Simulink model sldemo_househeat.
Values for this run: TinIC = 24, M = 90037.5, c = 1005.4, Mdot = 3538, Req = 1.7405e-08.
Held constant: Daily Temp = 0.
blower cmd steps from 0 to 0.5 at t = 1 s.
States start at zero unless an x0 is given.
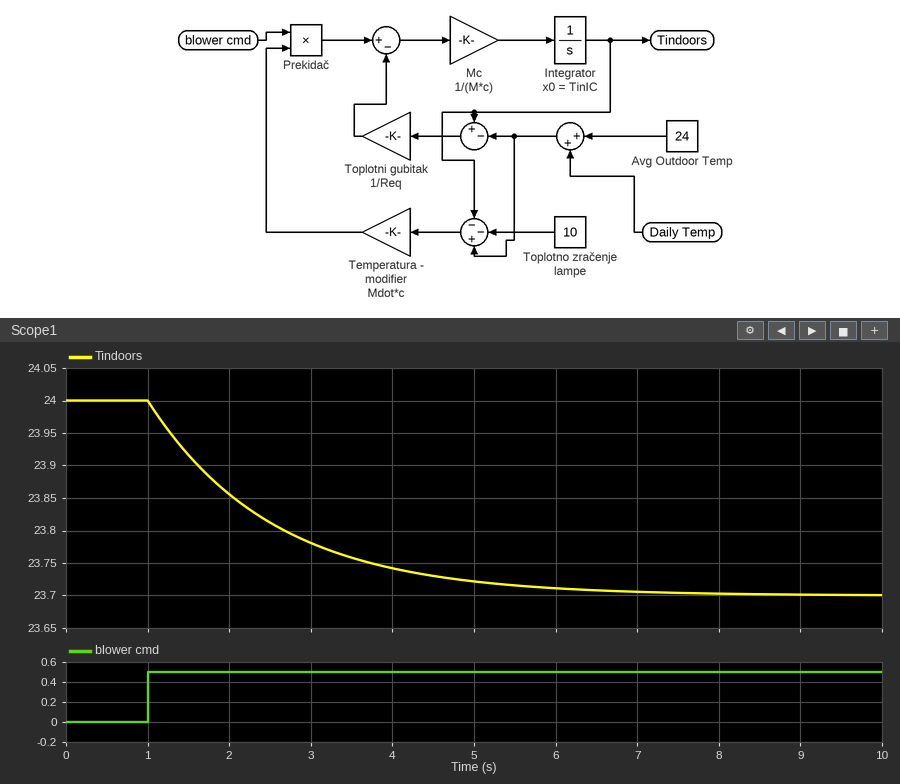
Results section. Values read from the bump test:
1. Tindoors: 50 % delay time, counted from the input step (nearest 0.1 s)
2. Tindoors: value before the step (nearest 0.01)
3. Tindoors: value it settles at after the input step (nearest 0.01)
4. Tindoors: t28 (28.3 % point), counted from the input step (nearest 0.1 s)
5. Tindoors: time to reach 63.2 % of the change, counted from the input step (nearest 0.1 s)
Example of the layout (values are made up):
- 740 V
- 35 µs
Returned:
- 1.1 s
- 24.00
- 23.70
- 0.5 s
- 1.5 s
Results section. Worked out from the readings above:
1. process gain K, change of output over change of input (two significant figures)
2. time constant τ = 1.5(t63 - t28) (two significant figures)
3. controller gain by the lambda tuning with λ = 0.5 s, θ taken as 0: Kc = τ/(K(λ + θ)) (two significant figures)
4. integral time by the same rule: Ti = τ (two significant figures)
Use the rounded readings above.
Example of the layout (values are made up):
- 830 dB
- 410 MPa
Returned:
- -0.60
- 1.5 s
- -5.0
- 1.5 s
